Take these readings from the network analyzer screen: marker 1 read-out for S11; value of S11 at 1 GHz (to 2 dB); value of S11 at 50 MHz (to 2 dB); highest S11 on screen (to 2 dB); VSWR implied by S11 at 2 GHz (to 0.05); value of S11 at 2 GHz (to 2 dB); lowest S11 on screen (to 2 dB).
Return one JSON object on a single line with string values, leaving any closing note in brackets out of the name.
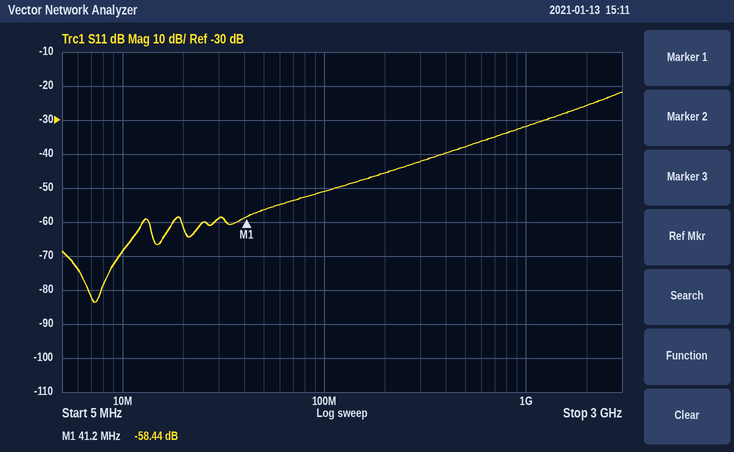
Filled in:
{"marker 1 read-out for S11": "-58.44 dB", "value of S11 at 1 GHz": "-32 dB", "value of S11 at 50 MHz": "-56 dB", "highest S11 on screen": "-22 dB", "VSWR implied by S11 at 2 GHz": "1.10", "value of S11 at 2 GHz": "-26 dB", "lowest S11 on screen": "-84 dB"}
